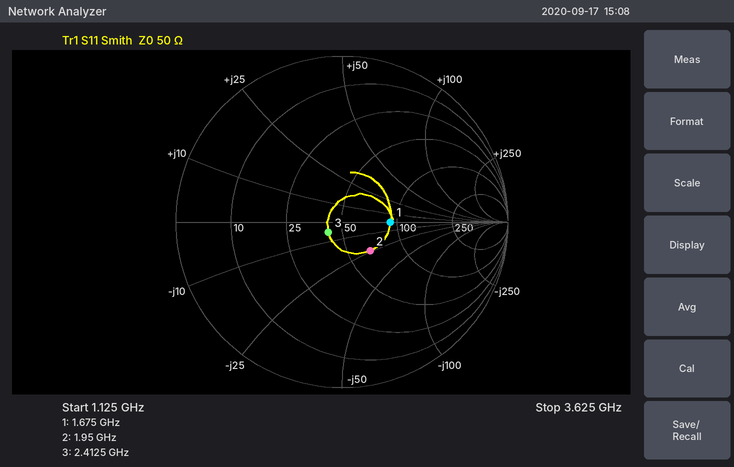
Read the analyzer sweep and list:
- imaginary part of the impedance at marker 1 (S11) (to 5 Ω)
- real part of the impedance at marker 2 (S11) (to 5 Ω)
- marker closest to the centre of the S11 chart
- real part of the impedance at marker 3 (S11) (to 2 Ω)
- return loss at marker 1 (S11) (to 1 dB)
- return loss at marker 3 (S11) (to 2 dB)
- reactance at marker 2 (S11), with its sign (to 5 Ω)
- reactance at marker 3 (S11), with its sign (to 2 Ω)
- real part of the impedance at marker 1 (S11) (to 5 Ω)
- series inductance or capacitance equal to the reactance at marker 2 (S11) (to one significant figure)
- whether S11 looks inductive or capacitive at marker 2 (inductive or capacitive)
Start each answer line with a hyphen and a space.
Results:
- 0 Ω
- 65 Ω
- marker 3
- 42 Ω
- 11 dB
- 20 dB
- -25 Ω
- -6 Ω
- 90 Ω
- 3 pF
- capacitive
